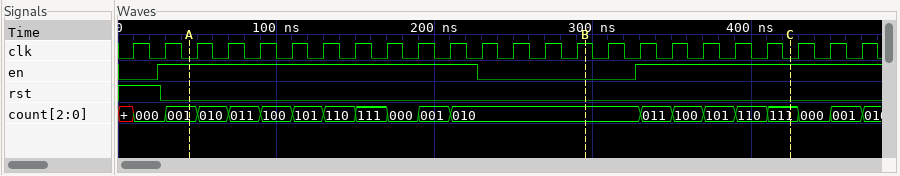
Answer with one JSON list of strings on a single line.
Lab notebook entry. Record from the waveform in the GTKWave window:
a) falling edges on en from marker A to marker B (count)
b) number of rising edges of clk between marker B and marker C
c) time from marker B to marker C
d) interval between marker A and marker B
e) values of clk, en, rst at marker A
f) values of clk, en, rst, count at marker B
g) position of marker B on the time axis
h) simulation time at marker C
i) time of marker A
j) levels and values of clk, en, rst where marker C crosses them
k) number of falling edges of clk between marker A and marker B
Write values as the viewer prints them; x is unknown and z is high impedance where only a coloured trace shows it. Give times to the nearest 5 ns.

["1", "6", "130 ns", "250 ns", "clk=0, en=1, rst=0", "clk=1, en=0, rst=0, count=010", "295 ns", "425 ns", "45 ns", "clk=0, en=1, rst=0", "12"]
